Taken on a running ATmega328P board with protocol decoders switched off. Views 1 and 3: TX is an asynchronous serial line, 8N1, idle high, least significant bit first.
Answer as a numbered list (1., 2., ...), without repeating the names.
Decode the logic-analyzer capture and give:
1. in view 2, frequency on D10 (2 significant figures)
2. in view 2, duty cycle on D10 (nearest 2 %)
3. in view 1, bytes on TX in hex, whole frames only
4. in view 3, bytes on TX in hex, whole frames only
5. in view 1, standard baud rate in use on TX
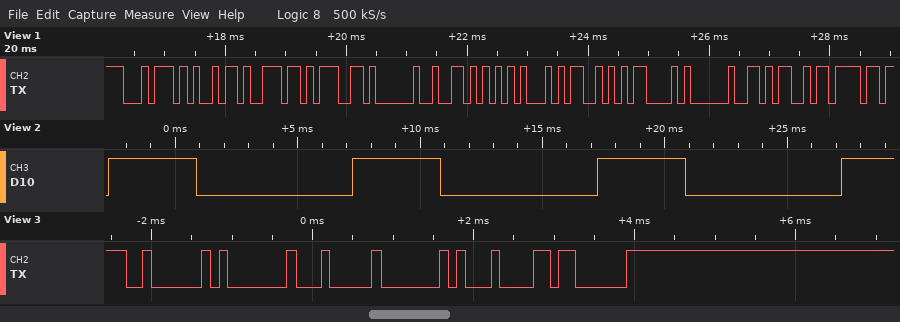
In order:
1. 100 Hz
2. 36 %
3. 74 69 6E 67 20 56 45 53 43 20 4D 6F
4. 02 01 04 40 84 03
5. 9600 baud
